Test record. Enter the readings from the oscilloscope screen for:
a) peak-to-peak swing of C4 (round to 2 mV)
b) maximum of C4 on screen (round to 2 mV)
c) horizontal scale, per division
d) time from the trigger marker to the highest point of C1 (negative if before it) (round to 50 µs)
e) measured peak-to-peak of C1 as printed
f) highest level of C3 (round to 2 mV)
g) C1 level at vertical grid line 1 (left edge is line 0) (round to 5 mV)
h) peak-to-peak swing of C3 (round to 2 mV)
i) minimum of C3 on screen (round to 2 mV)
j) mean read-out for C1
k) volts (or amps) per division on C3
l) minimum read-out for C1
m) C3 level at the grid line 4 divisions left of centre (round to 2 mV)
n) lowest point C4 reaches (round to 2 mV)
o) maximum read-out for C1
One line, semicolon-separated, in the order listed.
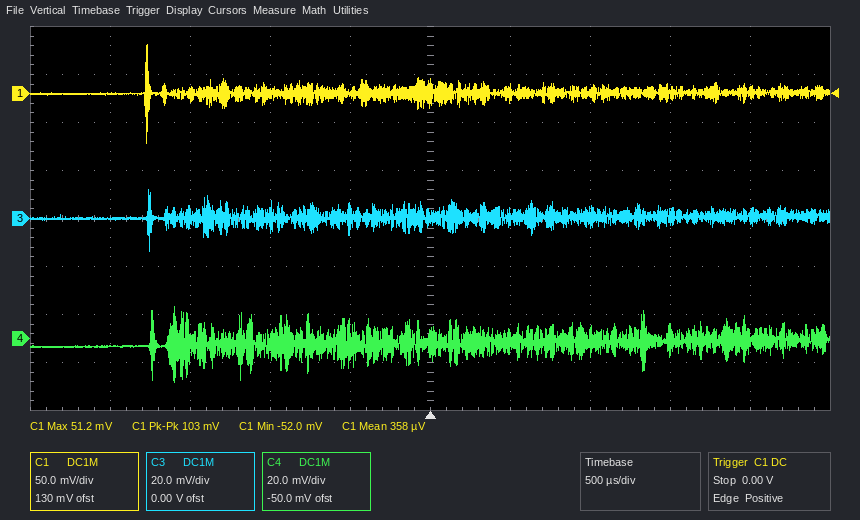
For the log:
32 mV; 14 mV; 500 µs; -1.75 ms; 103 mV; 12 mV; 0 mV; 26 mV; -14 mV; 358 µV; 20 mV; -52.0 mV; 0 mV; -18 mV; 51.2 mV
